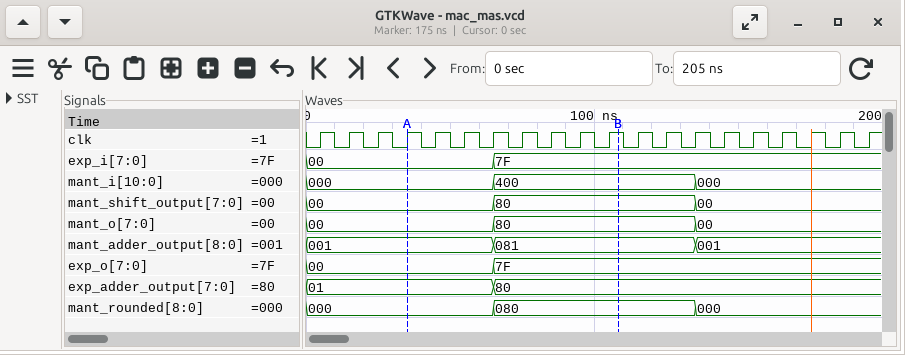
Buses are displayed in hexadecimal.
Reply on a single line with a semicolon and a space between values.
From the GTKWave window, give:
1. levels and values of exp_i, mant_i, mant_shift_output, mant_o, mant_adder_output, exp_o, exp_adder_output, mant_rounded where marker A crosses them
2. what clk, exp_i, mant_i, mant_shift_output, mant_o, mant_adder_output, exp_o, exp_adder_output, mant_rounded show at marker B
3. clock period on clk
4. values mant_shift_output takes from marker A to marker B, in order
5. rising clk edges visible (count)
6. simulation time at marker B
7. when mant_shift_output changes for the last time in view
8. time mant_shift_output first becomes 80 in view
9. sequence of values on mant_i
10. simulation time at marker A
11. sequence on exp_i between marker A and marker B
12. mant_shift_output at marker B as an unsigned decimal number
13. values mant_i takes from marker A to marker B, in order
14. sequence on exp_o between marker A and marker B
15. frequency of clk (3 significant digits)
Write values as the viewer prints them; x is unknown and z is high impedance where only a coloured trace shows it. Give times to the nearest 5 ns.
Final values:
exp_i=00, mant_i=000, mant_shift_output=00, mant_o=00, mant_adder_output=001, exp_o=00, exp_adder_output=01, mant_rounded=000; clk=1, exp_i=7F, mant_i=400, mant_shift_output=80, mant_o=80, mant_adder_output=081, exp_o=7F, exp_adder_output=80, mant_rounded=080; 10 ns; 00, 80; 20; 110 ns; 135 ns; 65 ns; 000, 400, 000; 35 ns; 00, 7F; 128; 000, 400; 00, 7F; 100 MHz
